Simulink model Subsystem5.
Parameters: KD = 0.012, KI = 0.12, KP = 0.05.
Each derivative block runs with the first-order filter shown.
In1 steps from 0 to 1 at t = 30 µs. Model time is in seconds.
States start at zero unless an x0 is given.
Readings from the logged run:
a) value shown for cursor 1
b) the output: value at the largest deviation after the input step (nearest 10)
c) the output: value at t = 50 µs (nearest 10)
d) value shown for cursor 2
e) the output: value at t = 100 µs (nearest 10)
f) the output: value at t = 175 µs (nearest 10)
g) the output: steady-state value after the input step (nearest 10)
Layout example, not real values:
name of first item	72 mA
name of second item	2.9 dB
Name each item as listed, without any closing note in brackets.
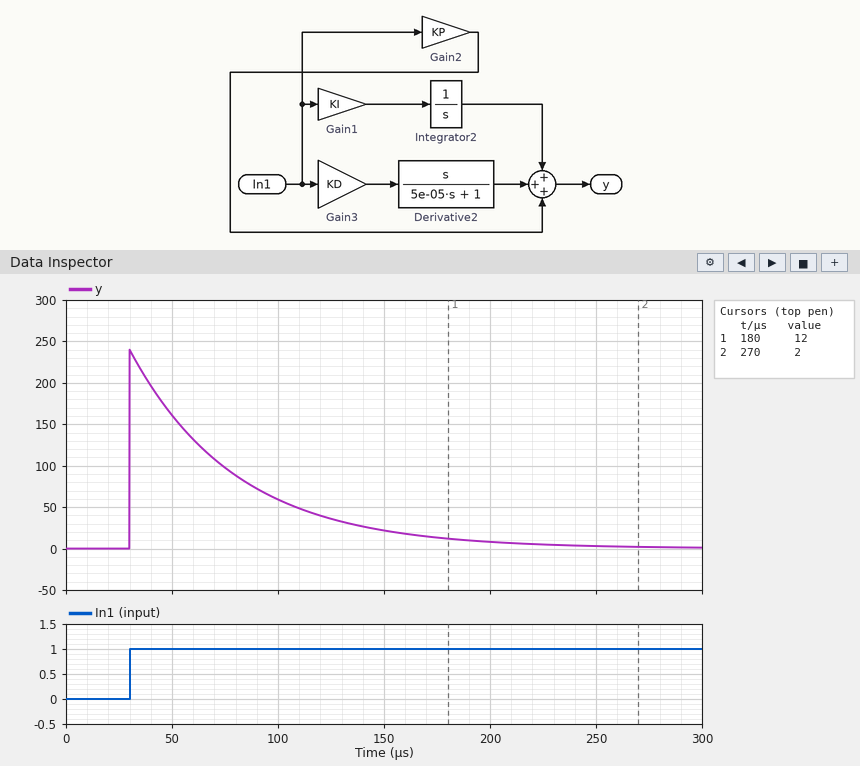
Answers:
value shown for cursor 1	12
the output: value at the largest deviation after the input step	240
the output: value at t = 50 µs	160
value shown for cursor 2	2
the output: value at t = 100 µs	60
the output: value at t = 175 µs	10
the output: steady-state value after the input step	0
